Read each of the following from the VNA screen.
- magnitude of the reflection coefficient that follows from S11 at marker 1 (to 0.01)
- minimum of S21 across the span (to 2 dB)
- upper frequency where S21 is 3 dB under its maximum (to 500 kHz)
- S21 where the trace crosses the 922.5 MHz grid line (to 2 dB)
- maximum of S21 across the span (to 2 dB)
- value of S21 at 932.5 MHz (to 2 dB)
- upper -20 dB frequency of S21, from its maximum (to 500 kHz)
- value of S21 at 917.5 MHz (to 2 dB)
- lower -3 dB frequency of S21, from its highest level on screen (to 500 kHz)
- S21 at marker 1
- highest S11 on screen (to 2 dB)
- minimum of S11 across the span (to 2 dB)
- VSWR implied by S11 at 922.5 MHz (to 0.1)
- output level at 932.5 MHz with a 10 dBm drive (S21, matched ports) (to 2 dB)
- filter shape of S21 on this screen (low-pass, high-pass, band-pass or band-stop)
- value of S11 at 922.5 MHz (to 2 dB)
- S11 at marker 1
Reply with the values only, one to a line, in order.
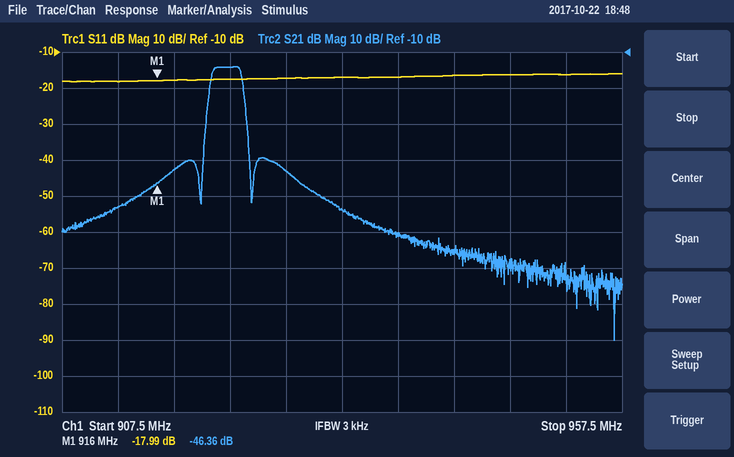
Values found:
0.13
-90 dB
923.5 MHz
-14 dB
-14 dB
-54 dB
924.0 MHz
-42 dB
921.0 MHz
-46.36 dB
-16 dB
-18 dB
1.3
-44 dBm
band-pass
-18 dB
-17.99 dB
